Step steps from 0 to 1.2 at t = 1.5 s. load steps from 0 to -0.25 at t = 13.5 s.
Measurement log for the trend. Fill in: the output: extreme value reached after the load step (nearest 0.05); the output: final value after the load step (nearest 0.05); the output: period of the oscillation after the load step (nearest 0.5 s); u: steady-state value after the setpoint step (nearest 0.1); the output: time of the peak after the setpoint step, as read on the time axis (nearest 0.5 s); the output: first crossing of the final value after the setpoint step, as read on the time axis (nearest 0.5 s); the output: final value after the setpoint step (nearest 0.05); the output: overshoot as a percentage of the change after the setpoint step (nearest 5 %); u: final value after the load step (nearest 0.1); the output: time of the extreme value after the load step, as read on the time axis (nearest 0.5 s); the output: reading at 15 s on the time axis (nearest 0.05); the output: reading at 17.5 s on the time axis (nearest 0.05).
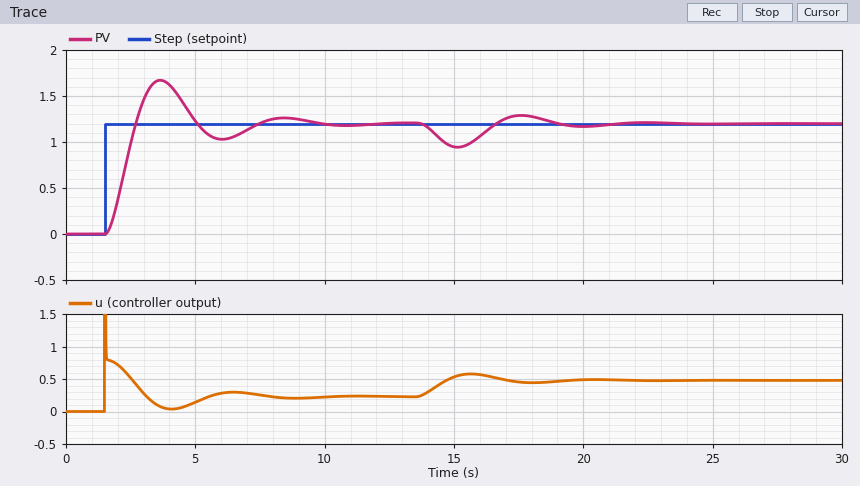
0.95
1.20
5.0 s
0.2
3.5 s
2.5 s
1.20
40 %
0.5
15.0 s
0.95
1.30
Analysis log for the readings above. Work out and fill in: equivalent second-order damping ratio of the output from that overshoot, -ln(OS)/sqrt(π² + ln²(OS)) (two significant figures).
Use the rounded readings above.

0.28
